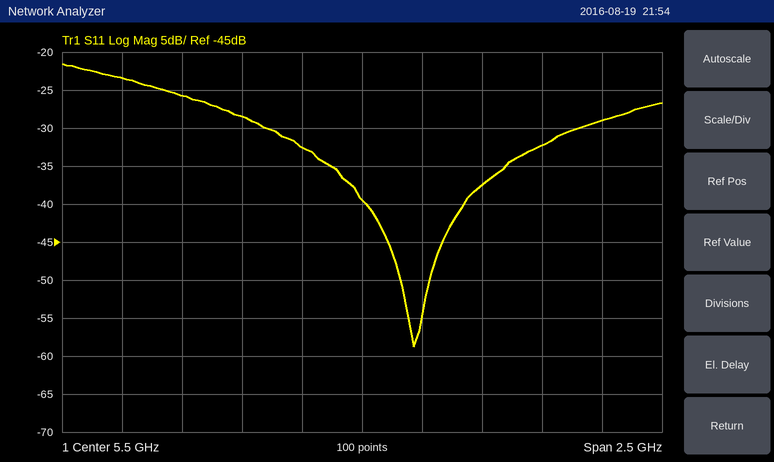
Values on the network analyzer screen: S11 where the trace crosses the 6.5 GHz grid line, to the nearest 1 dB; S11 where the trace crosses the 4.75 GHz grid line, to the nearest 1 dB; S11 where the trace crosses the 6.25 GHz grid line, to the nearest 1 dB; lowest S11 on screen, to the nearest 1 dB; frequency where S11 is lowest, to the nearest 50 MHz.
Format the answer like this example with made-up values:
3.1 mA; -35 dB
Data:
-29 dB; -26 dB; -32 dB; -59 dB; 5.70 GHz
